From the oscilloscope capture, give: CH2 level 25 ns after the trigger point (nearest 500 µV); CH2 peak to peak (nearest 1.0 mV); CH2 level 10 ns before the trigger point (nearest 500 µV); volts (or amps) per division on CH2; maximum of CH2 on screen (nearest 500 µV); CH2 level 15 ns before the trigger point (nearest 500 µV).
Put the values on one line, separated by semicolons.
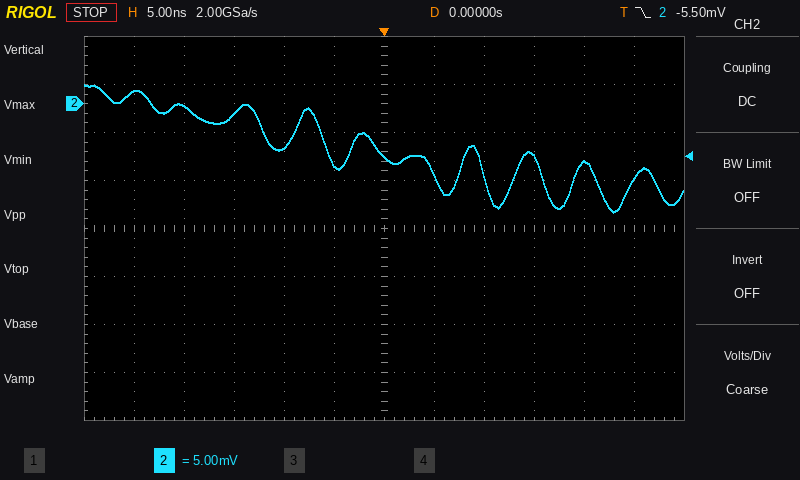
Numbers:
-8.0 mV; 13.0 mV; -4.5 mV; 5 mV; 2.0 mV; -1.0 mV
